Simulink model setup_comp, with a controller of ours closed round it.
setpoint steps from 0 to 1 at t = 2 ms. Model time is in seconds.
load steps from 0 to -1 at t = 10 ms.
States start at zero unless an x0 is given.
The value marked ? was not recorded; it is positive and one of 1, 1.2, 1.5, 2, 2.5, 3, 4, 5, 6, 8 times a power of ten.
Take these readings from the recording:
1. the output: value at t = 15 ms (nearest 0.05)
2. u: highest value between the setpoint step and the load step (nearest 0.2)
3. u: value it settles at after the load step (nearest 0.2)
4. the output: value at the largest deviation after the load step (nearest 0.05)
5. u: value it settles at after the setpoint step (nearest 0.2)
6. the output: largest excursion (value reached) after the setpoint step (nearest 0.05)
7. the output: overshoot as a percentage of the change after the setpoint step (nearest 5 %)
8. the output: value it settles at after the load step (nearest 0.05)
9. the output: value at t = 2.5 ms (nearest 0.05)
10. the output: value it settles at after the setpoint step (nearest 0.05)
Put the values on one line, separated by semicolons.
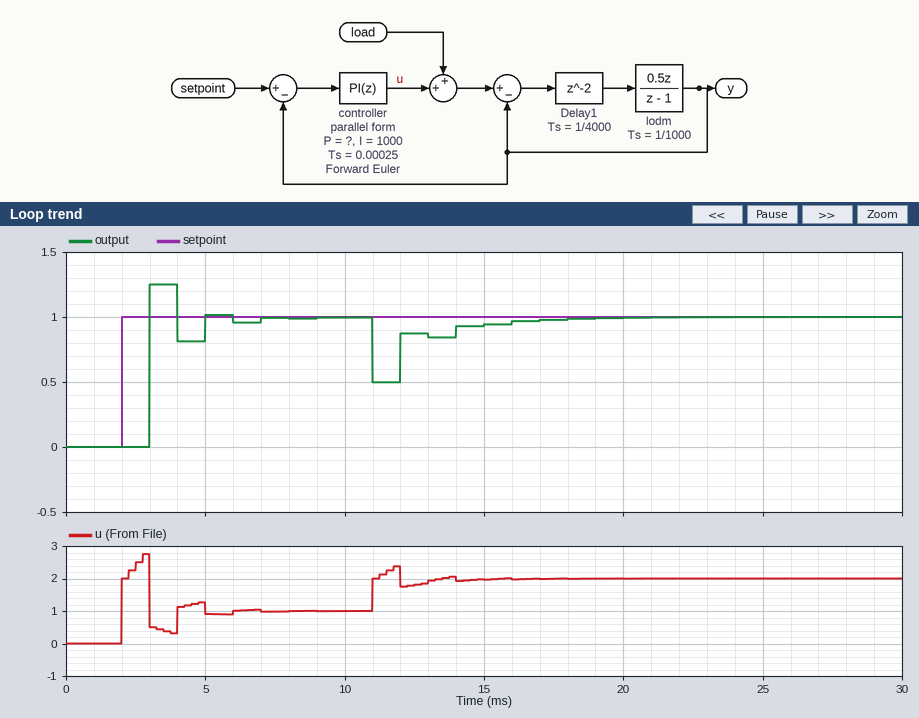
0.95; 2.8; 2.0; 0.50; 1.0; 1.25; 25 %; 1.00; 0.00; 1.00
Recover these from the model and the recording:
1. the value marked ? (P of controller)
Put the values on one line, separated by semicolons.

2
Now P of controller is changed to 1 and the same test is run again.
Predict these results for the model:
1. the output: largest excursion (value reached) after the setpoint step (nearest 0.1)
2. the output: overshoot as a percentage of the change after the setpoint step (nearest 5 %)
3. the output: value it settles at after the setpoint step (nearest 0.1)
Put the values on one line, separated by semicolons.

1.1; 10 %; 1.0
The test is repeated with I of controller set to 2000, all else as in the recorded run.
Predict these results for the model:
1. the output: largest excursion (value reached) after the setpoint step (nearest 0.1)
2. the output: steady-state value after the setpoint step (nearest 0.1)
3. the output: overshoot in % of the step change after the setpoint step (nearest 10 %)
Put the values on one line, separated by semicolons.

1.5; 1.0; 50 %
